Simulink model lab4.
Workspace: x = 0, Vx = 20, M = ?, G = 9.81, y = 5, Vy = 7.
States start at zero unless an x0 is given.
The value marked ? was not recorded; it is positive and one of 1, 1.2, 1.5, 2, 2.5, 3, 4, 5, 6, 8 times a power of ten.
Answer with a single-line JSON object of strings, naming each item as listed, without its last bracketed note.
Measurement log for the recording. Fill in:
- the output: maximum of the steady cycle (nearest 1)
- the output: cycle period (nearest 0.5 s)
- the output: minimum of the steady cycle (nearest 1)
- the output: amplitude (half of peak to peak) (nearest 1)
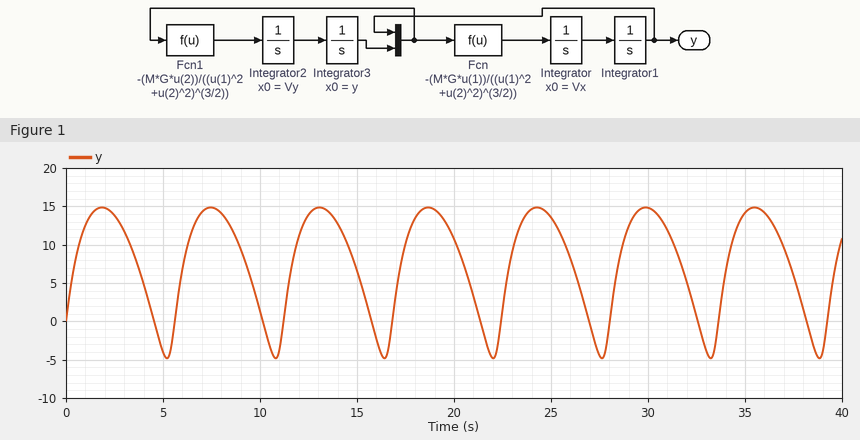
{"the output: maximum of the steady cycle": "15", "the output: cycle period": "5.5 s", "the output: minimum of the steady cycle": "-5", "the output: amplitude (half of peak to peak)": "10"}
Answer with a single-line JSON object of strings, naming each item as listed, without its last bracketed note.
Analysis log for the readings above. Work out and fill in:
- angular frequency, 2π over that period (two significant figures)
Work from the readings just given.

{"angular frequency, 2π over that period": "1.1 rad/s"}
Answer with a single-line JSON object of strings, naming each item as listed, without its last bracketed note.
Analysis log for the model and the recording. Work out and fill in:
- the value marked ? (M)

{"the value marked ?": "150"}
